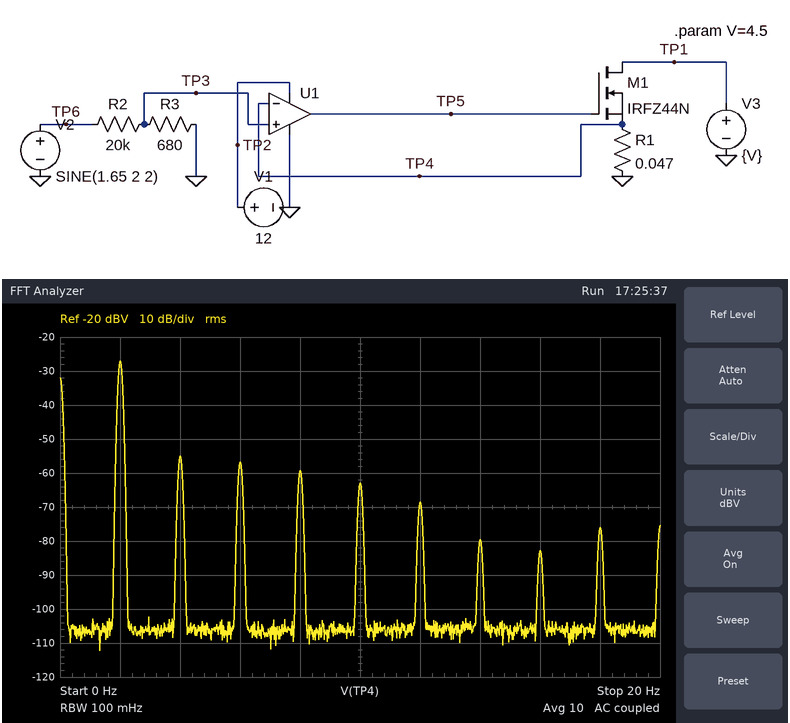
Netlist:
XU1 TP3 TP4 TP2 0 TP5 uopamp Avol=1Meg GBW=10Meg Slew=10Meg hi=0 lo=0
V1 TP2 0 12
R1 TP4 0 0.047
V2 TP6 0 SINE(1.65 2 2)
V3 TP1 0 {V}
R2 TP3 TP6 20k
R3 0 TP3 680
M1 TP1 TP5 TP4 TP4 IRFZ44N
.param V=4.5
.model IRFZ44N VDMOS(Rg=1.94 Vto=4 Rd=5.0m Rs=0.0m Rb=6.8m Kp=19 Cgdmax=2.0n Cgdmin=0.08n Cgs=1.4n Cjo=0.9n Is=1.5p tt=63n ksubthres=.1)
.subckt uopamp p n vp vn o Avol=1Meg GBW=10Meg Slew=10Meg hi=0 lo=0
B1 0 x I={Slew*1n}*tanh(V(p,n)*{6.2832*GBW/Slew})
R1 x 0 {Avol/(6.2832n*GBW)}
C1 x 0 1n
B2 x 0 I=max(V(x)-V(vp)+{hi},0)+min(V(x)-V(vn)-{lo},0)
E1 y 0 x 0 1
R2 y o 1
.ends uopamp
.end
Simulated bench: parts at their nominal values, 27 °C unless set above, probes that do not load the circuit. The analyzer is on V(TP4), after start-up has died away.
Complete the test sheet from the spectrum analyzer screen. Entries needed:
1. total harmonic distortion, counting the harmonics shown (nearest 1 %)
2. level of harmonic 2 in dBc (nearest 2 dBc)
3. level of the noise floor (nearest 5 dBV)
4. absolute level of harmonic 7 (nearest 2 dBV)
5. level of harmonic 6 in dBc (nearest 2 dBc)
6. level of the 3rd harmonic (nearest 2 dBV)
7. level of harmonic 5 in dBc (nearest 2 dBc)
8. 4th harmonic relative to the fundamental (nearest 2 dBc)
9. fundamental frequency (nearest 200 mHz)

6 %
-28 dBc
-105 dBV
-80 dBV
-42 dBc
-56 dBV
-36 dBc
-32 dBc
2.0 Hz
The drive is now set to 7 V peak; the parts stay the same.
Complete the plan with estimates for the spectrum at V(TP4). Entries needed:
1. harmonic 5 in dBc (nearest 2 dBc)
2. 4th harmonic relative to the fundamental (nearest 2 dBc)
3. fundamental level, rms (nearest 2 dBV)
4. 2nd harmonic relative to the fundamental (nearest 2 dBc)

-28 dBc
-28 dBc
-20 dBV
-10 dBc
